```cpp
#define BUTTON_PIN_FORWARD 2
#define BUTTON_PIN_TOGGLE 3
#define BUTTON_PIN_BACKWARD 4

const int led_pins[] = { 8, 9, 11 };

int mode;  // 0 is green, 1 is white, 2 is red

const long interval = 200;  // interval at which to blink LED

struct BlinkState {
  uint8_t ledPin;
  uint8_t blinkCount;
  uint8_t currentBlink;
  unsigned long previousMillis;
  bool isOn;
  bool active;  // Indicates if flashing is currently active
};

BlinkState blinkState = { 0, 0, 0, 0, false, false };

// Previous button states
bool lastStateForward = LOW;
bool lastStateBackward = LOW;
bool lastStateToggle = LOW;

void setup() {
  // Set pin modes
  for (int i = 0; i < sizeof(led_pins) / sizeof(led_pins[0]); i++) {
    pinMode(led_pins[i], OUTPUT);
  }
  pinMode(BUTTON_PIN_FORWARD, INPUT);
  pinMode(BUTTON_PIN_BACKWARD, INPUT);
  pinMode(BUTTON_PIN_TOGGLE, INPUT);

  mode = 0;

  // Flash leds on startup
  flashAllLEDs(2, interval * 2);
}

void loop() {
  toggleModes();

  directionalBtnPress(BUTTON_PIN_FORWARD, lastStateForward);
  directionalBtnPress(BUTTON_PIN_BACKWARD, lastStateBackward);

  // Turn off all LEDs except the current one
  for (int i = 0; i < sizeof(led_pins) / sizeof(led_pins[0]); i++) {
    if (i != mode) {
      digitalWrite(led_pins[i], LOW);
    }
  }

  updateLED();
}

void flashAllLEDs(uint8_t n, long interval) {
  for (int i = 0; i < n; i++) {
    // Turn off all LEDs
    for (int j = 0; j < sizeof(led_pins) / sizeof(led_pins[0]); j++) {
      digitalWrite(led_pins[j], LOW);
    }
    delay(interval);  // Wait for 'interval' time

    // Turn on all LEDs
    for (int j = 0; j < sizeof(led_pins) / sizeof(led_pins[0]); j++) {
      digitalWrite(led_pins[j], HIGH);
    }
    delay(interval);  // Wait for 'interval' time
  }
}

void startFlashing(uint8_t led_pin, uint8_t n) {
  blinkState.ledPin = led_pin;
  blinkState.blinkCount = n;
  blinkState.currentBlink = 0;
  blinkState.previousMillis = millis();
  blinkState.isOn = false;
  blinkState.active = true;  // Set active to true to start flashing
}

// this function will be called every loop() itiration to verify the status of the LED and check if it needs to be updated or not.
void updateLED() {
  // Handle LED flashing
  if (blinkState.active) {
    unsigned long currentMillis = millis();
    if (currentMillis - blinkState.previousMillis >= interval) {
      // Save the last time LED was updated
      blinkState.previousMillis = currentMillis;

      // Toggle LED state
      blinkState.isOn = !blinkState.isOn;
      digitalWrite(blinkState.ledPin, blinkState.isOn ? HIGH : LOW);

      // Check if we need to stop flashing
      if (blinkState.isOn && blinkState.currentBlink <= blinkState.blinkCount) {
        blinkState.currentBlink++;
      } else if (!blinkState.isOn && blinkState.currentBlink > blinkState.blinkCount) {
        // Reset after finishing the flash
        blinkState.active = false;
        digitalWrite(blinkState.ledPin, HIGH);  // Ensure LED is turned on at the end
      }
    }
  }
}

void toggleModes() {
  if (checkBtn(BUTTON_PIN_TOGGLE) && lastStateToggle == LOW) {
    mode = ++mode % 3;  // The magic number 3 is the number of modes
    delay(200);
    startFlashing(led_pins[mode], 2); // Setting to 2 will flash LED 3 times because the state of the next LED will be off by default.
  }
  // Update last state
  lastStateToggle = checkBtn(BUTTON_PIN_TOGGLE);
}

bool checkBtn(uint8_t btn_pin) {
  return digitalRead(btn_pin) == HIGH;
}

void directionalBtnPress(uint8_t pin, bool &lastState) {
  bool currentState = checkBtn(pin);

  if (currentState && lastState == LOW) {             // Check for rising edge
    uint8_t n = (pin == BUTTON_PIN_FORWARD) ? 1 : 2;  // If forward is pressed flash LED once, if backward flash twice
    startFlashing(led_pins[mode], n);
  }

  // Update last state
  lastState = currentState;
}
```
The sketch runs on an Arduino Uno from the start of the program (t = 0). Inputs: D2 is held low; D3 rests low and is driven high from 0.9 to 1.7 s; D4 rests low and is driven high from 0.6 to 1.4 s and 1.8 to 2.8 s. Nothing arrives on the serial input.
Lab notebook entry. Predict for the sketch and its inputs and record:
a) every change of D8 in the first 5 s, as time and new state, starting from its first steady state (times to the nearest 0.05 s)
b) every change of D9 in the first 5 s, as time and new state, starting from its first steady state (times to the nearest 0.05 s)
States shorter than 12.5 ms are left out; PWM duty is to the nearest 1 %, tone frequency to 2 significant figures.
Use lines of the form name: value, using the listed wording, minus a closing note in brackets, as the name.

every change of D8 in the first 5 s, as time and new state, starting from its first steady state: 0 s low; 0.4 s high; 0.8 s low; 1.2 s high; 1.8 s low
every change of D9 in the first 5 s, as time and new state, starting from its first steady state: 0 s low; 0.4 s high; 0.8 s low; 1.2 s high; 2.2 s low; 2.4 s high; 2.6 s low; 2.8 s high
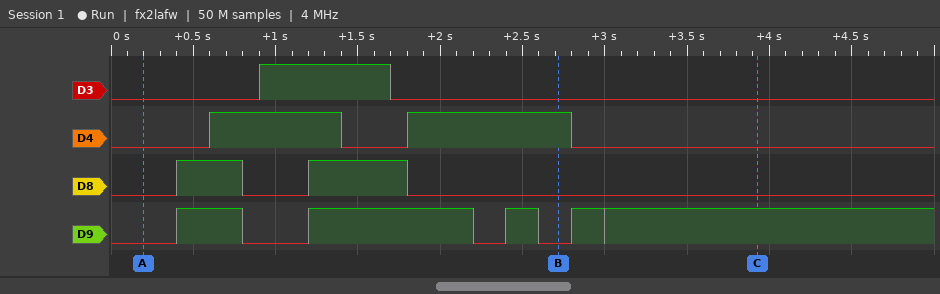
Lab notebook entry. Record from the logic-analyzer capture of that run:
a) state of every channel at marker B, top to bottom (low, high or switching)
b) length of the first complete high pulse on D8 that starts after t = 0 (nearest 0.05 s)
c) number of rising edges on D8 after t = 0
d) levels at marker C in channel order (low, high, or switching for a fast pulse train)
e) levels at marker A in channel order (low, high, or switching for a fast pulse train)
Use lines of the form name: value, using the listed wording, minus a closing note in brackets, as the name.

state of every channel at marker B, top to bottom: D3 low, D4 high, D8 low, D9 low
length of the first complete high pulse on D8 that starts after t = 0: 0.40 s
number of rising edges on D8 after t = 0: 2
levels at marker C in channel order: D3 low, D4 low, D8 low, D9 high
levels at marker A in channel order: D3 low, D4 low, D8 low, D9 low
